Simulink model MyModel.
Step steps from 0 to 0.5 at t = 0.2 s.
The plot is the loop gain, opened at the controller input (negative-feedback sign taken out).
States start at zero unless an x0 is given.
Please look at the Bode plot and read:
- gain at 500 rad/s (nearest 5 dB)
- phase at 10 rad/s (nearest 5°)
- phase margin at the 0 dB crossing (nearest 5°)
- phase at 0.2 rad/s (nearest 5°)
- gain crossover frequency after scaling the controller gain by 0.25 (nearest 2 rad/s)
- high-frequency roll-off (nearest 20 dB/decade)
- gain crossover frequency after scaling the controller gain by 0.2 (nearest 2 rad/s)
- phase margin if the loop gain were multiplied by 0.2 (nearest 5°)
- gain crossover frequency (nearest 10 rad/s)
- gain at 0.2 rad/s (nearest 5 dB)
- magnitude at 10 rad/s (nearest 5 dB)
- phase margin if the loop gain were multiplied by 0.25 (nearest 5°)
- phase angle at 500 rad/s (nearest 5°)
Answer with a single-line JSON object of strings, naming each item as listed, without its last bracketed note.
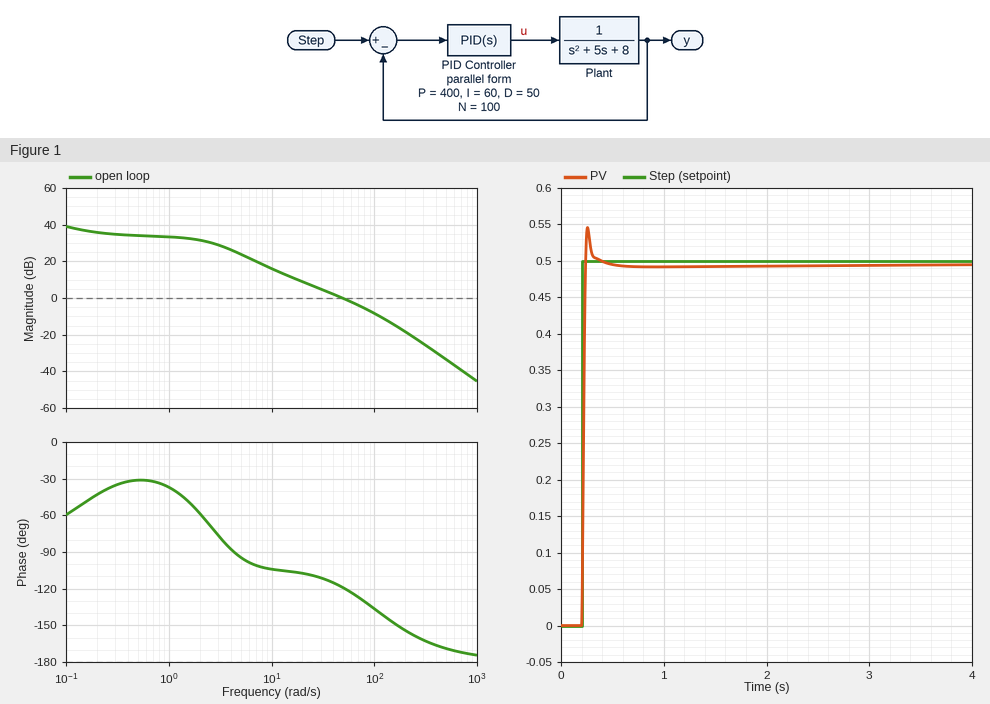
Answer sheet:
{"gain at 500 rad/s": "-35 dB", "phase at 10 rad/s": "-105°", "phase margin at the 0 dB crossing": "60°", "phase at 0.2 rad/s": "-45°", "gain crossover frequency after scaling the controller gain by 0.25": "14 rad/s", "high-frequency roll-off": "-40 dB/decade", "gain crossover frequency after scaling the controller gain by 0.2": "12 rad/s", "phase margin if the loop gain were multiplied by 0.2": "75°", "gain crossover frequency": "50 rad/s", "gain at 0.2 rad/s": "35 dB", "magnitude at 10 rad/s": "15 dB", "phase margin if the loop gain were multiplied by 0.25": "75°", "phase angle at 500 rad/s": "-170°"}
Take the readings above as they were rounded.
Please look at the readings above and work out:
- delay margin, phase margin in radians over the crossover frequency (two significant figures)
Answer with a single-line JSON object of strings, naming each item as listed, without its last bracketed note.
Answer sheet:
{"delay margin, phase margin in radians over the crossover frequency": "0.021 s"}
